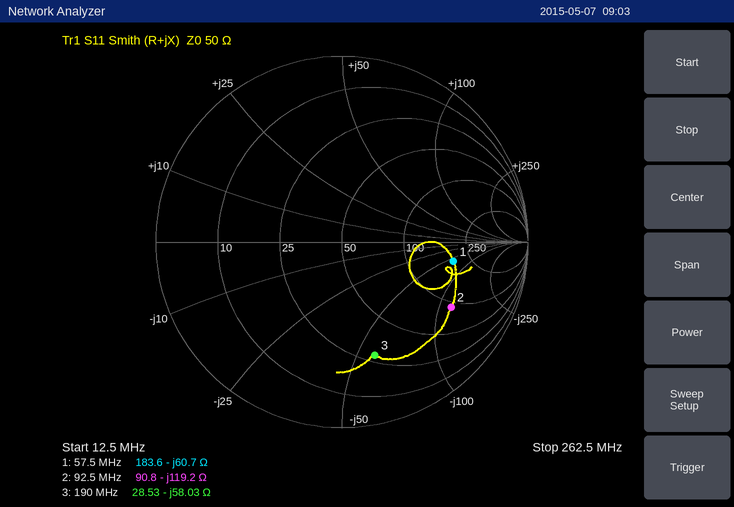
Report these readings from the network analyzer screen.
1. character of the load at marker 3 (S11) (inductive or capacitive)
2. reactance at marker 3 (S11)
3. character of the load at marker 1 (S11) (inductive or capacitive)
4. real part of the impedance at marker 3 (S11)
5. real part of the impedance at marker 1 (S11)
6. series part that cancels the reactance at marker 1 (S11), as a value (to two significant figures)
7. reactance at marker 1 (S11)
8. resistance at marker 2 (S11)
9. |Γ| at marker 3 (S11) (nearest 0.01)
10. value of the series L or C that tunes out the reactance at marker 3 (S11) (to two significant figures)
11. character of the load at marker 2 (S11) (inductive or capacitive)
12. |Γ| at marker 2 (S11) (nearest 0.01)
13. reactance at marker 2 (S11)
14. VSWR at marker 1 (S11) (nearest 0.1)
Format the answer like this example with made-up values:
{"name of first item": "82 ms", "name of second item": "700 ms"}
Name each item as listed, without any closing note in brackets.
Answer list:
{"character of the load at marker 3 (S11)": "capacitive", "reactance at marker 3": "-58.03 Ω", "character of the load at marker 1 (S11)": "capacitive", "real part of the impedance at marker 3": "28.53 Ω", "real part of the impedance at marker 1": "183.6 Ω", "series part that cancels the reactance at marker 1 (S11), as a value": "170 nH", "reactance at marker 1": "-60.7 Ω", "resistance at marker 2": "90.8 Ω", "|Γ| at marker 3 (S11)": "0.63", "value of the series L or C that tunes out the reactance at marker 3 (S11)": "49 nH", "character of the load at marker 2 (S11)": "capacitive", "|Γ| at marker 2 (S11)": "0.68", "reactance at marker 2": "-119.2 Ω", "VSWR at marker 1 (S11)": "4.1"}
